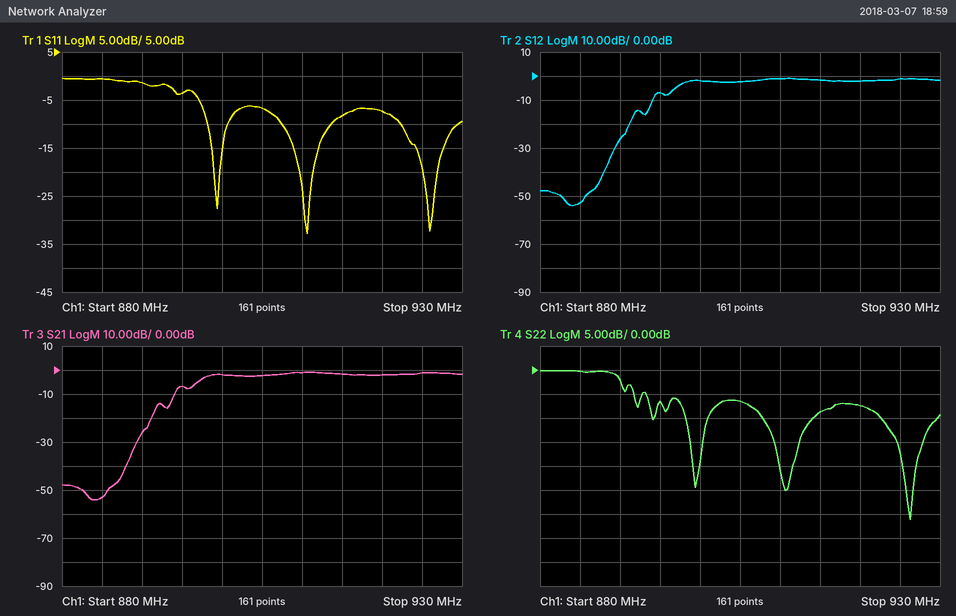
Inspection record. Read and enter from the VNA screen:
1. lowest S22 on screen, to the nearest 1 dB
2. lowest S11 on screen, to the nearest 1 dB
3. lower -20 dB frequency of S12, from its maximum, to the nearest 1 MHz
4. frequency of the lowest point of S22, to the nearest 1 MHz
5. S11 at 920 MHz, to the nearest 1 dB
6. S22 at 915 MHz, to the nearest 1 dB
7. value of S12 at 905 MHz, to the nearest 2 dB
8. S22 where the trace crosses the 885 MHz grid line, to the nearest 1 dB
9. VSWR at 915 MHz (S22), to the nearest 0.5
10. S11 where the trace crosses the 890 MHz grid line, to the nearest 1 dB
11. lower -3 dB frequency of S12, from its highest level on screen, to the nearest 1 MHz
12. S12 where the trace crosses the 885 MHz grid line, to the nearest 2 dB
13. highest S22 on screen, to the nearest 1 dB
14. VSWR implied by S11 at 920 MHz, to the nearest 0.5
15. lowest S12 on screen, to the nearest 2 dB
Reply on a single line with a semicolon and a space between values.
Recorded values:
-31 dB; -33 dB; 891 MHz; 926 MHz; -7 dB; -9 dB; -2 dB; 0 dB; 2.0; -1 dB; 897 MHz; -52 dB; 0 dB; 2.5; -54 dB
